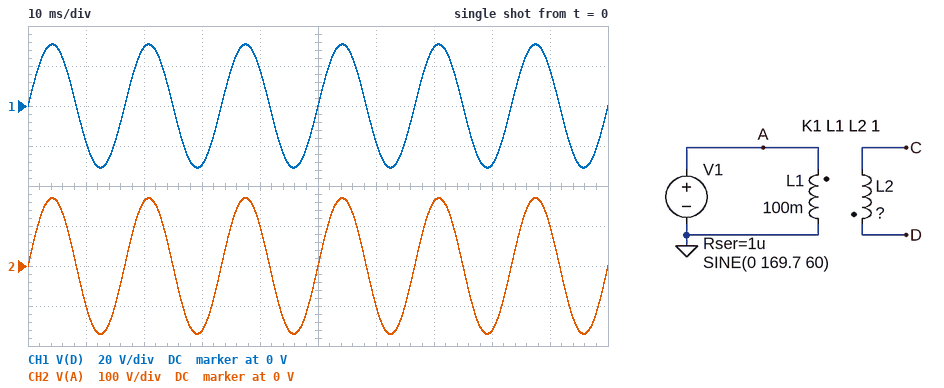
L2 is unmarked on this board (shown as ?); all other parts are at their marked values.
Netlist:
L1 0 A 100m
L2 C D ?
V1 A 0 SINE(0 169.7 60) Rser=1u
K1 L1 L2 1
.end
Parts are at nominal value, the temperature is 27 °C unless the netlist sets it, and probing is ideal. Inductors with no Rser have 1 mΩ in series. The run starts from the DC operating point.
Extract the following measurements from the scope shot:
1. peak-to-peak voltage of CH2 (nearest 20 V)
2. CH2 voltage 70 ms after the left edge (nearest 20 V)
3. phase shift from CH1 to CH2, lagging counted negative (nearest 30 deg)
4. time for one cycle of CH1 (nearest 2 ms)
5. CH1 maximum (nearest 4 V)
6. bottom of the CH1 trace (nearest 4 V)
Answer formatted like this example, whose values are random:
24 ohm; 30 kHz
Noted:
340 V; 160 V; 0 deg; 16 ms; 32 V; -32 V
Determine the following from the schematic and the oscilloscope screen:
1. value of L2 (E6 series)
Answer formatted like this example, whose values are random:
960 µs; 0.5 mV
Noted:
3.3 mH
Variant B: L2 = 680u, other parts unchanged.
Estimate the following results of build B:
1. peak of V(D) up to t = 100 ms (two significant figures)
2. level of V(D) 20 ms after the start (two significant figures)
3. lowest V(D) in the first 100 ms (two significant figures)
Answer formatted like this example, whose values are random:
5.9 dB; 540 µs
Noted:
14 V; 13 V; -14 V
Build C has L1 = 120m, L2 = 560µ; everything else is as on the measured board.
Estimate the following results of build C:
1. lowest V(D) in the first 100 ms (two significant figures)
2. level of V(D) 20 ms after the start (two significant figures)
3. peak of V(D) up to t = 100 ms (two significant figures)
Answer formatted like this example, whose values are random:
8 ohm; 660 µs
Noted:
-12 V; 11 V; 12 V
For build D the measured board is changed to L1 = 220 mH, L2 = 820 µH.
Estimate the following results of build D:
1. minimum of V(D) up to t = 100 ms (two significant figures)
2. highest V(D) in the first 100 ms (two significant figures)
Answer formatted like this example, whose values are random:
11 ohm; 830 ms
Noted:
-10 V; 10 V
